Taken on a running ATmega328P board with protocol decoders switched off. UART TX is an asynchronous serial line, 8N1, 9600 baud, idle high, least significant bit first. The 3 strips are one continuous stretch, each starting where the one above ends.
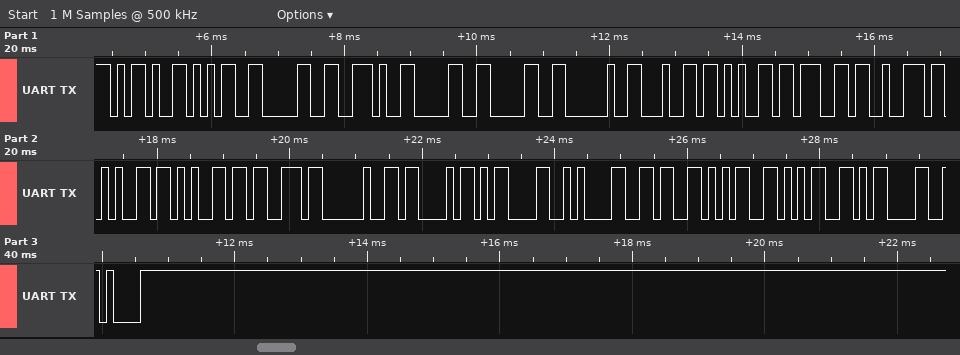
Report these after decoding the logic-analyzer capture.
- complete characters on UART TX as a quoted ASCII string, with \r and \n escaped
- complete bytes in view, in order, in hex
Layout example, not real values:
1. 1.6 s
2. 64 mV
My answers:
1. "-50.00 degrees C\r\n655\r\n"
2. 2D 35 30 2E 30 30 20 64 65 67 72 65 65 73 20 43 0D 0A 36 35 35 0D 0A
